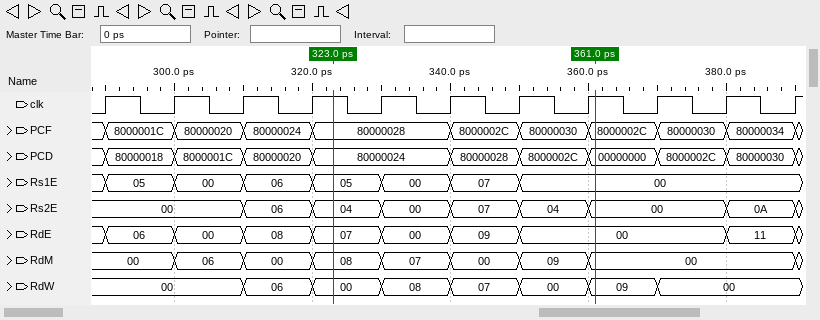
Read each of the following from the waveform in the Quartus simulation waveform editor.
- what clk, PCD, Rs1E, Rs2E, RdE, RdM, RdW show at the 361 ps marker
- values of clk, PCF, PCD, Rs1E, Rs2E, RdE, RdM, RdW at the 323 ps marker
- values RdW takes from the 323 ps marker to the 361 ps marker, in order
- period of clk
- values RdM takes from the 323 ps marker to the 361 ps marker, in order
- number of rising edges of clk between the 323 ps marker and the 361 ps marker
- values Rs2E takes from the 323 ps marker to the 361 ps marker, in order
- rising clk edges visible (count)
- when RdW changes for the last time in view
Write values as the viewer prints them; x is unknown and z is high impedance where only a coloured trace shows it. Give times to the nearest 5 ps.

clk=1, PCD=00000000, Rs1E=00, Rs2E=00, RdE=00, RdM=00, RdW=09
clk=1, PCF=80000028, PCD=80000024, Rs1E=05, Rs2E=04, RdE=07, RdM=08, RdW=00
00, 08, 07, 00, 09
10 ps
08, 07, 00, 09, 00
4
04, 00, 07, 04, 00
11
370 ps
